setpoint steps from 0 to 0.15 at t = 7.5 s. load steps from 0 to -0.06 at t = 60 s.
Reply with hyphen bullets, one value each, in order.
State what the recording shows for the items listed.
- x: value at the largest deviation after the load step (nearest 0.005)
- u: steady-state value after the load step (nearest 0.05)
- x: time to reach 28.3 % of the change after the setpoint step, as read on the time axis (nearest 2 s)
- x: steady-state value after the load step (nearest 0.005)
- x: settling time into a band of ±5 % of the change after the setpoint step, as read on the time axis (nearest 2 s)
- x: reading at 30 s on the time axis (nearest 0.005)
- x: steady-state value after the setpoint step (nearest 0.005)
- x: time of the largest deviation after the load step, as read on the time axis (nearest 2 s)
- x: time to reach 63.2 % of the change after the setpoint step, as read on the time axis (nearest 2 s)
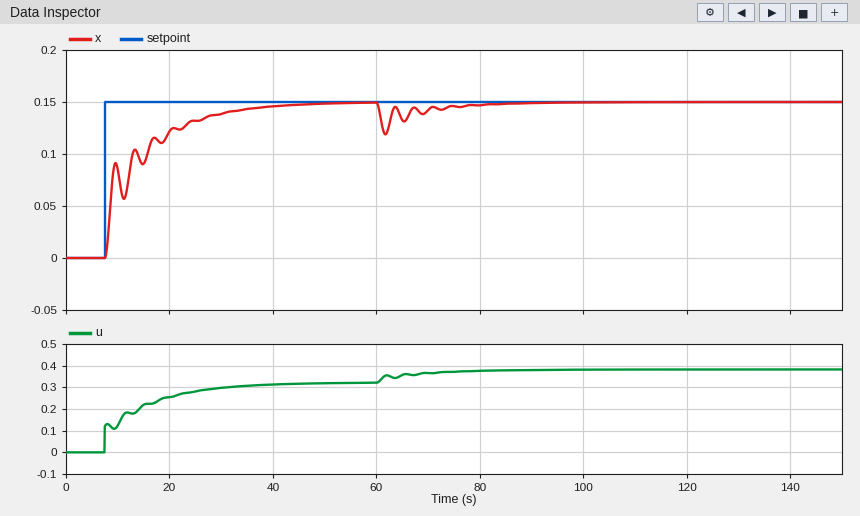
- 0.120
- 0.40
- 8 s
- 0.150
- 34 s
- 0.140
- 0.150
- 62 s
- 12 s
